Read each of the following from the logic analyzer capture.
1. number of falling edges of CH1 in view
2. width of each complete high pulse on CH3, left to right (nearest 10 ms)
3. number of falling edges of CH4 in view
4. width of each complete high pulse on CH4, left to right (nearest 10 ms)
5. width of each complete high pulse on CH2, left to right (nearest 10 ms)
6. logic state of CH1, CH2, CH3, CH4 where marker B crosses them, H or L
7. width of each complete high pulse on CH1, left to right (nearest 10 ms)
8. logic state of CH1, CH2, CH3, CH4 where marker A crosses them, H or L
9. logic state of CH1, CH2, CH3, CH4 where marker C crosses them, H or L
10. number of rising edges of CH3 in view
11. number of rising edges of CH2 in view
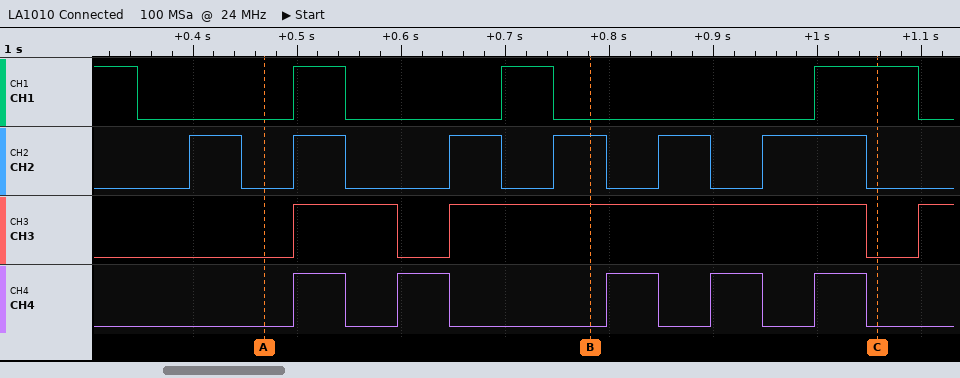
4
100 ms, 400 ms
5
50 ms, 50 ms, 50 ms, 50 ms, 50 ms
50 ms, 50 ms, 50 ms, 50 ms, 50 ms, 100 ms
CH1=L, CH2=H, CH3=H, CH4=L
50 ms, 50 ms, 100 ms
CH1=L, CH2=L, CH3=L, CH4=L
CH1=H, CH2=L, CH3=L, CH4=L
3
6
